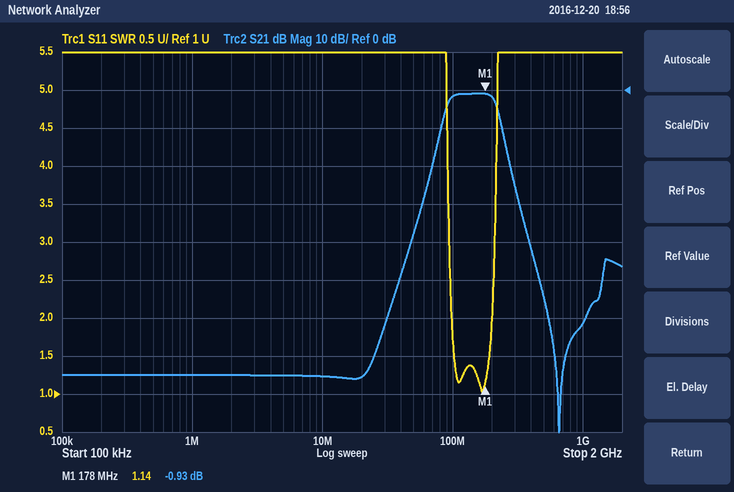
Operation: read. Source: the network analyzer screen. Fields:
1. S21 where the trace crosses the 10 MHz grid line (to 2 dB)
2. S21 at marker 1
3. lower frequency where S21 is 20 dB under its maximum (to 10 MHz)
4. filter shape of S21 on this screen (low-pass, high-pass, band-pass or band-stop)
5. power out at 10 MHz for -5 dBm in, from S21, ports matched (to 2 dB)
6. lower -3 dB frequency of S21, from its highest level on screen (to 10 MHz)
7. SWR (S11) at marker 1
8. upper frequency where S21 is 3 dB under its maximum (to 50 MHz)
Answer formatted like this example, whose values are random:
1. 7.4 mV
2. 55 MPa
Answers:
1. -76 dB
2. -0.93 dB
3. 70 MHz
4. band-pass
5. -80 dBm
6. 90 MHz
7. 1.14
8. 200 MHz
